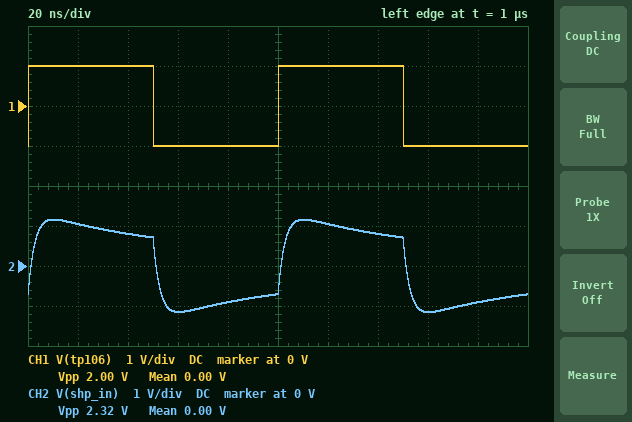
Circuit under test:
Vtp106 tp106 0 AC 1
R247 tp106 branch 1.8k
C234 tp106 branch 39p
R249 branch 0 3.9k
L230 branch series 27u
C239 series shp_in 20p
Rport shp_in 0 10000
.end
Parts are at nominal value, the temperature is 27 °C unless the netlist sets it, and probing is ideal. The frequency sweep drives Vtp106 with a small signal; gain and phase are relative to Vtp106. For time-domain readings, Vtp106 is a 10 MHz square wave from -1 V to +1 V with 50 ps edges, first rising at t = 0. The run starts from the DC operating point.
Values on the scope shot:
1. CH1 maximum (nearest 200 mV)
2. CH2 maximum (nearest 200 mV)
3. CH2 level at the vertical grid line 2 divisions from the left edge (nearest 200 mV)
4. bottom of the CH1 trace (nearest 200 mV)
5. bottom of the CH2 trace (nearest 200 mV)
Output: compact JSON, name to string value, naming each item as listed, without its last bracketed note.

{"CH1 maximum": "1.0 V", "CH2 maximum": "1.2 V", "CH2 level at the vertical grid line 2 divisions from the left edge": "800 mV", "bottom of the CH1 trace": "-1.0 V", "bottom of the CH2 trace": "-1.2 V"}
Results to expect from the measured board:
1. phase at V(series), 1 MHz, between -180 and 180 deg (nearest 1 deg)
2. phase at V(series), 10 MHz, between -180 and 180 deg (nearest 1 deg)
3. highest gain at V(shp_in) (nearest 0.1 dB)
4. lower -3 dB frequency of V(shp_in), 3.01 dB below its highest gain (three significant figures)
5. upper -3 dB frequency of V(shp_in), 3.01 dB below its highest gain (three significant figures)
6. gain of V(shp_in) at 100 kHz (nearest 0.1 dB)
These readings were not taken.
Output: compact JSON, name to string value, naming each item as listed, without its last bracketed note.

{"phase at V(series), 1 MHz, between -180 and 180 deg": "5 deg", "phase at V(series), 10 MHz, between -180 and 180 deg": "-2 deg", "highest gain at V(shp_in)": "-0.3 dB", "lower -3 dB frequency of V(shp_in), 3.01 dB below its highest gain": "2.15 MHz", "upper -3 dB frequency of V(shp_in), 3.01 dB below its highest gain": "63.7 MHz", "gain of V(shp_in) at 100 kHz": "-21.4 dB"}
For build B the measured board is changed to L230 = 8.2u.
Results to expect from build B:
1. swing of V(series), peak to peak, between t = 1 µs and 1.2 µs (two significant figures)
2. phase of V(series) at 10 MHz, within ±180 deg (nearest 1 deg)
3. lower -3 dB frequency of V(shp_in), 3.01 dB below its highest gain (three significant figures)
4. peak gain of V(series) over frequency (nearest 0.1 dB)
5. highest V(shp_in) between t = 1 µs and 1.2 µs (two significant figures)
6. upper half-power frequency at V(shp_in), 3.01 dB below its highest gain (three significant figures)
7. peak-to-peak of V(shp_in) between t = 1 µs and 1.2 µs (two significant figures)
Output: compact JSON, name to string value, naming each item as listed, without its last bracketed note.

{"swing of V(series), peak to peak, between t = 1 µs and 1.2 µs": "2.3 V", "phase of V(series) at 10 MHz, within ±180 deg": "5 deg", "lower -3 dB frequency of V(shp_in), 3.01 dB below its highest gain": "2.35 MHz", "peak gain of V(series) over frequency": "-0.1 dB", "highest V(shp_in) between t = 1 µs and 1.2 µs": "1.3 V", "upper half-power frequency at V(shp_in), 3.01 dB below its highest gain": "199 MHz", "peak-to-peak of V(shp_in) between t = 1 µs and 1.2 µs": "2.5 V"}
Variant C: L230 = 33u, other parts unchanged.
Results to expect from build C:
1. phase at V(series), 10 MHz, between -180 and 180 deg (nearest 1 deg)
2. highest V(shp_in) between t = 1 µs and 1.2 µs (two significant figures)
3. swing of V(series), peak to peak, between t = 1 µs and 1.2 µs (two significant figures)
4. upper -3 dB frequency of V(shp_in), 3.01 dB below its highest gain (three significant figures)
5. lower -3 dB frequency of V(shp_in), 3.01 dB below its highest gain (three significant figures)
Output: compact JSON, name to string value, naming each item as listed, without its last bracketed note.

{"phase at V(series), 10 MHz, between -180 and 180 deg": "-4 deg", "highest V(shp_in) between t = 1 µs and 1.2 µs": "1.1 V", "swing of V(series), peak to peak, between t = 1 µs and 1.2 µs": "2.1 V", "upper -3 dB frequency of V(shp_in), 3.01 dB below its highest gain": "53.0 MHz", "lower -3 dB frequency of V(shp_in), 3.01 dB below its highest gain": "2.09 MHz"}
